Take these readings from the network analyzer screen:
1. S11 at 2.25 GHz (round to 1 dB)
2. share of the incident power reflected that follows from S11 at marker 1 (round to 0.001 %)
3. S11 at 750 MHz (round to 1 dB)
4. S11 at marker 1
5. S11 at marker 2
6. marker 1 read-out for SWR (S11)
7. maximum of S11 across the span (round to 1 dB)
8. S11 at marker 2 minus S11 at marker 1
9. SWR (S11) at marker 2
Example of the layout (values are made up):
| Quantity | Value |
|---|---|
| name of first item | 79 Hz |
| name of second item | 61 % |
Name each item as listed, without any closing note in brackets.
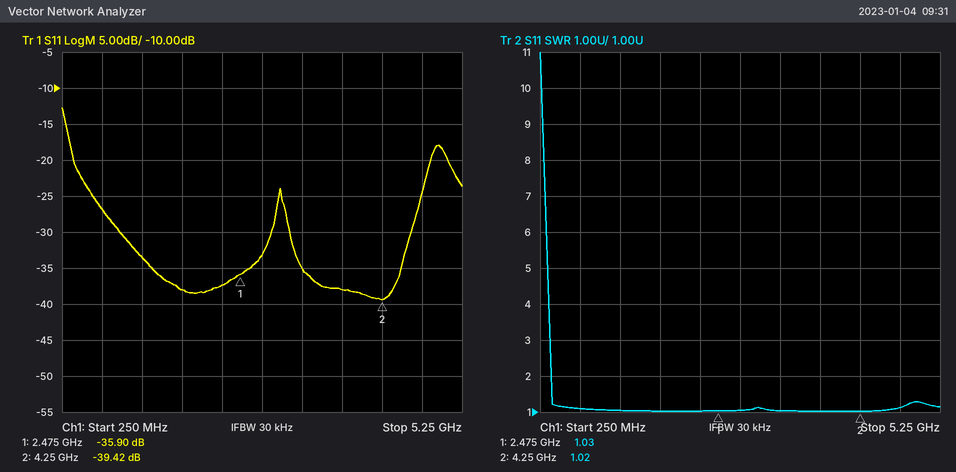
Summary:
| Quantity | Value |
|---|---|
| S11 at 2.25 GHz | -37 dB |
| share of the incident power reflected that follows from S11 at marker 1 | 0.026 % |
| S11 at 750 MHz | -27 dB |
| S11 at marker 1 | -35.90 dB |
| S11 at marker 2 | -39.42 dB |
| marker 1 read-out for SWR | 1.03 |
| maximum of S11 across the span | -13 dB |
| S11 at marker 2 minus S11 at marker 1 | -3.52 dB |
| SWR (S11) at marker 2 | 1.02 |
